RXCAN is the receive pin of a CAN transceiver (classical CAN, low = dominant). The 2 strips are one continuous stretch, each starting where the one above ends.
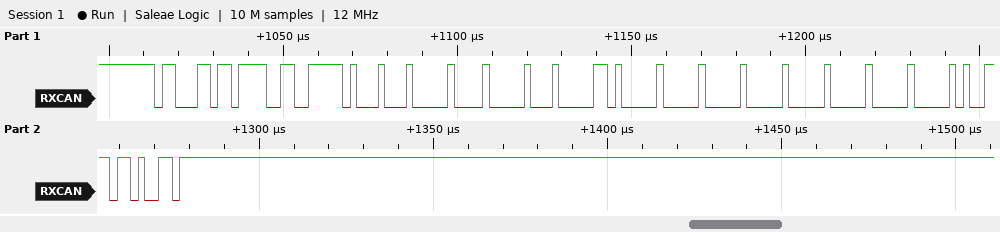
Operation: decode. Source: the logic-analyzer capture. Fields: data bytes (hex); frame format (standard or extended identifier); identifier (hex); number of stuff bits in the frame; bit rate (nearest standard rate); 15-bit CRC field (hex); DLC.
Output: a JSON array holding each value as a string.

["02 01 05 00 00 00 00 00", "extended", "0x18DB33F1", "12", "500 kbit/s", "0x2769", "8"]
